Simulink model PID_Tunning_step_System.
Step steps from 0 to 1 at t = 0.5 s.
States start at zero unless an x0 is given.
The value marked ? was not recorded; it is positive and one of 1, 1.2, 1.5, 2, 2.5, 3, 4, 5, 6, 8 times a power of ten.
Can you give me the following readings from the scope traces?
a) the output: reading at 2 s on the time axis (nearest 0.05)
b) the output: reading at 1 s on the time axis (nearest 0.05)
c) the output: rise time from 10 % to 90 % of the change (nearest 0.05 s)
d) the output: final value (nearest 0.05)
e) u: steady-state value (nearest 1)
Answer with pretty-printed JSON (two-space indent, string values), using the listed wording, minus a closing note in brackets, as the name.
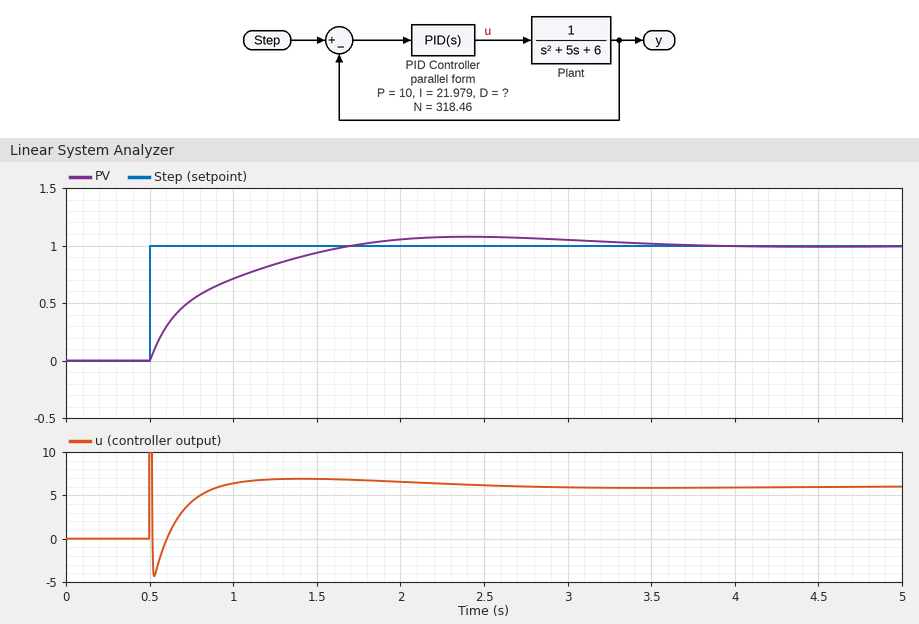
{
  "the output: reading at 2 s on the time axis": "1.05",
  "the output: reading at 1 s on the time axis": "0.70",
  "the output: rise time from 10 % to 90 % of the change": "0.85 s",
  "the output: final value": "1.00",
  "u: steady-state value": "6"
}
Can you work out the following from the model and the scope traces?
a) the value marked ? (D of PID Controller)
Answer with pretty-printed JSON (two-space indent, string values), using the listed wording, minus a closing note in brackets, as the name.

{
  "the value marked ?": "4"
}
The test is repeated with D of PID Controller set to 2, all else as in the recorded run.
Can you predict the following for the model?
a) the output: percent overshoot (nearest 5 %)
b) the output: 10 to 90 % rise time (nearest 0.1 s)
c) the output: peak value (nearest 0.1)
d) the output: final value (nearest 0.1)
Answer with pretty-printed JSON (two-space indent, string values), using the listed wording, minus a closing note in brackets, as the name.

{
  "the output: percent overshoot": "10 %",
  "the output: 10 to 90 % rise time": "0.7 s",
  "the output: peak value": "1.1",
  "the output: final value": "1.0"
}
